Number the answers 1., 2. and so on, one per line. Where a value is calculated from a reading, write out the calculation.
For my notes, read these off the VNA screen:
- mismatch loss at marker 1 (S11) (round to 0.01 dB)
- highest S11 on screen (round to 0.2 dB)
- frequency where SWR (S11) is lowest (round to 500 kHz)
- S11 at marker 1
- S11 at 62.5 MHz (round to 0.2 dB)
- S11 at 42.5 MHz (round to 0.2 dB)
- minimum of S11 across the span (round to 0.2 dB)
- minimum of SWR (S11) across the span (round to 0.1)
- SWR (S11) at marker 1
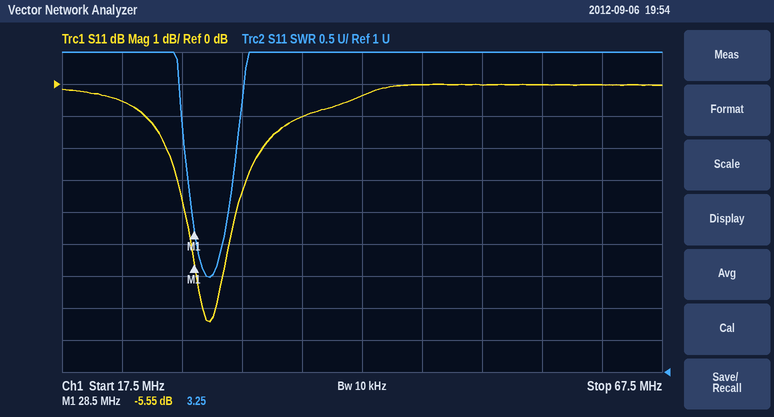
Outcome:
1. −10 log10(1 − 10^(-5.55/10)) ≈ 1.42 dB
2. 0.0 dB
3. 30.0 MHz
4. -5.55 dB
5. 0.0 dB
6. -0.4 dB
7. -7.4 dB
8. 2.5
9. 3.25
